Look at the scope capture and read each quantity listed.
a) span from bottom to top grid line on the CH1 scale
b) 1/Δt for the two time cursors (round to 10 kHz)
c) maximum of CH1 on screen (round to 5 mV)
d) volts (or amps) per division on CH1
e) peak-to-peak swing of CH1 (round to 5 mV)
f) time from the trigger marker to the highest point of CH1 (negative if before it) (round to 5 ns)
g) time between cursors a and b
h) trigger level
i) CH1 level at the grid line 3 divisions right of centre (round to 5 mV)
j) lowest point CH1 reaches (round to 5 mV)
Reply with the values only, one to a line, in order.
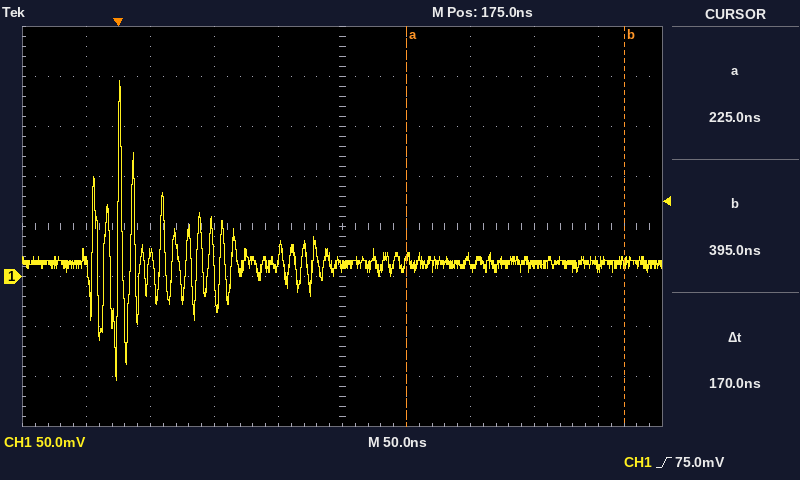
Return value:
400 mV
5.88 MHz
195 mV
50 mV
300 mV
0 ns
170 ns
75.0 mV
10 mV
-105 mV
